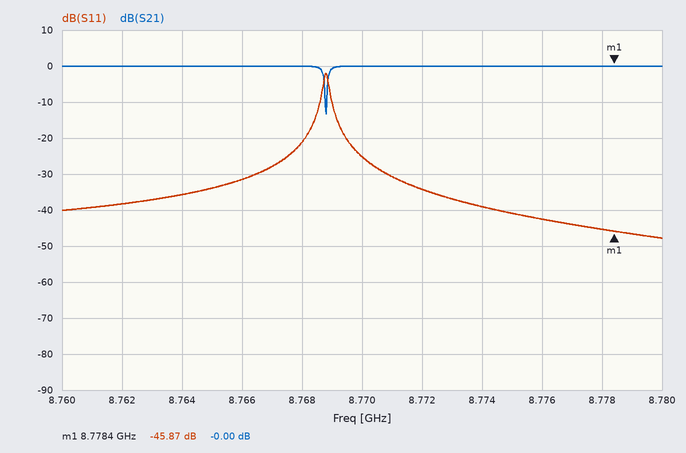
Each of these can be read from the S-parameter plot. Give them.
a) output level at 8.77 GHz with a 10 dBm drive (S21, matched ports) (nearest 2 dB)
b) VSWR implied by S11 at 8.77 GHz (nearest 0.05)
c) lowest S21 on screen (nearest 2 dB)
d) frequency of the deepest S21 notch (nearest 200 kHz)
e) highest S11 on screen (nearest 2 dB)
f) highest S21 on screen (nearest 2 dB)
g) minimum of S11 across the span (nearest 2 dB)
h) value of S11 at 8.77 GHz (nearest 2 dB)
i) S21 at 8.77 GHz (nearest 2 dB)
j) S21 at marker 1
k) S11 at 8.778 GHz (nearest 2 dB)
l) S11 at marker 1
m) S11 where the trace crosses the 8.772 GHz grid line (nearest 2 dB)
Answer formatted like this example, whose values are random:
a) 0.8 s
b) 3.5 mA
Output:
a) 10 dBm
b) 1.10
c) -14 dB
d) 8.7688 GHz
e) -2 dB
f) 0 dB
g) -48 dB
h) -26 dB
i) 0 dB
j) -0.00 dB
k) -46 dB
l) -45.87 dB
m) -34 dB
